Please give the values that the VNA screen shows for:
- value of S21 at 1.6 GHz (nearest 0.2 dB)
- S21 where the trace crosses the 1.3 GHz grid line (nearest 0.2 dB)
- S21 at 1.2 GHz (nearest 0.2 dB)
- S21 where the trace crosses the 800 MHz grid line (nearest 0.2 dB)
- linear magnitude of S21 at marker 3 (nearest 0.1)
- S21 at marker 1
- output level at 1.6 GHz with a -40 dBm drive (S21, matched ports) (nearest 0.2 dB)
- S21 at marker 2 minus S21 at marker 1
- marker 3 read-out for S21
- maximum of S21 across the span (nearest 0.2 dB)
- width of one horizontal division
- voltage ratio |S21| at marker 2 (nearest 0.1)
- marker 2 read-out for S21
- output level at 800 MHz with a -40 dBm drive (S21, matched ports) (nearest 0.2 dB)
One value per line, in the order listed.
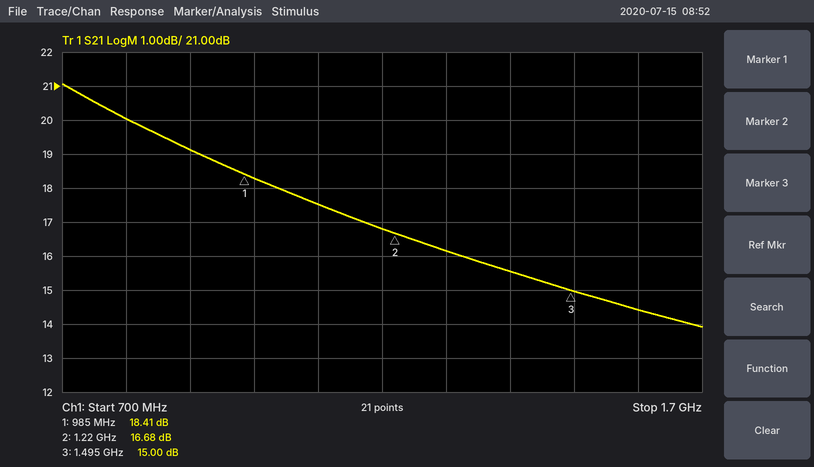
14.4 dB
16.2 dB
16.8 dB
20.0 dB
5.6
18.41 dB
-25.6 dBm
-1.73 dB
15.00 dB
21.0 dB
100 MHz
6.8
16.68 dB
-20.0 dBm
